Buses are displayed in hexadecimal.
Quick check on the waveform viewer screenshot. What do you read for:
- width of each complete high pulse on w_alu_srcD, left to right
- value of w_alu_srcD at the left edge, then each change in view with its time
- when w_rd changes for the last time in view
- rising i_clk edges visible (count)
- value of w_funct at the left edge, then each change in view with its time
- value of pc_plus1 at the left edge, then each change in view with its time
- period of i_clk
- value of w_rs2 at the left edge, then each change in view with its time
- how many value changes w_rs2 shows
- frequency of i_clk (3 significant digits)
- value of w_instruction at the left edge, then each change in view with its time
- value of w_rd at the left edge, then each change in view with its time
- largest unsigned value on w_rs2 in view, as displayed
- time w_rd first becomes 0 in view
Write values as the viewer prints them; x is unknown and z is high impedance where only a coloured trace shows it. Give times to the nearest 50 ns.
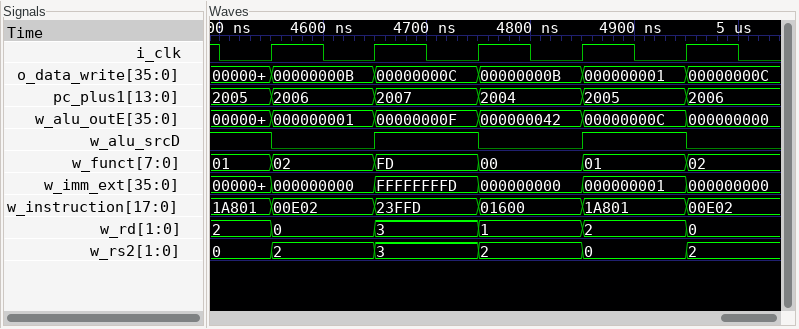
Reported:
100 ns, 100 ns
1, 0 at 4550 ns, 1 at 4650 ns, 0 at 4750 ns, 1 at 4850 ns, 0 at 4950 ns
4950 ns
5
01, 02 at 4550 ns, FD at 4650 ns, 00 at 4750 ns, 01 at 4850 ns, 02 at 4950 ns
2005, 2006 at 4550 ns, 2007 at 4650 ns, 2004 at 4750 ns, 2005 at 4850 ns, 2006 at 4950 ns
100 ns
0, 2 at 4550 ns, 3 at 4650 ns, 2 at 4750 ns, 0 at 4850 ns, 2 at 4950 ns
5
10.0 MHz
1A801, 00E02 at 4550 ns, 23FFD at 4650 ns, 01600 at 4750 ns, 1A801 at 4850 ns, 00E02 at 4950 ns
2, 0 at 4550 ns, 3 at 4650 ns, 1 at 4750 ns, 2 at 4850 ns, 0 at 4950 ns
3
4550 ns
